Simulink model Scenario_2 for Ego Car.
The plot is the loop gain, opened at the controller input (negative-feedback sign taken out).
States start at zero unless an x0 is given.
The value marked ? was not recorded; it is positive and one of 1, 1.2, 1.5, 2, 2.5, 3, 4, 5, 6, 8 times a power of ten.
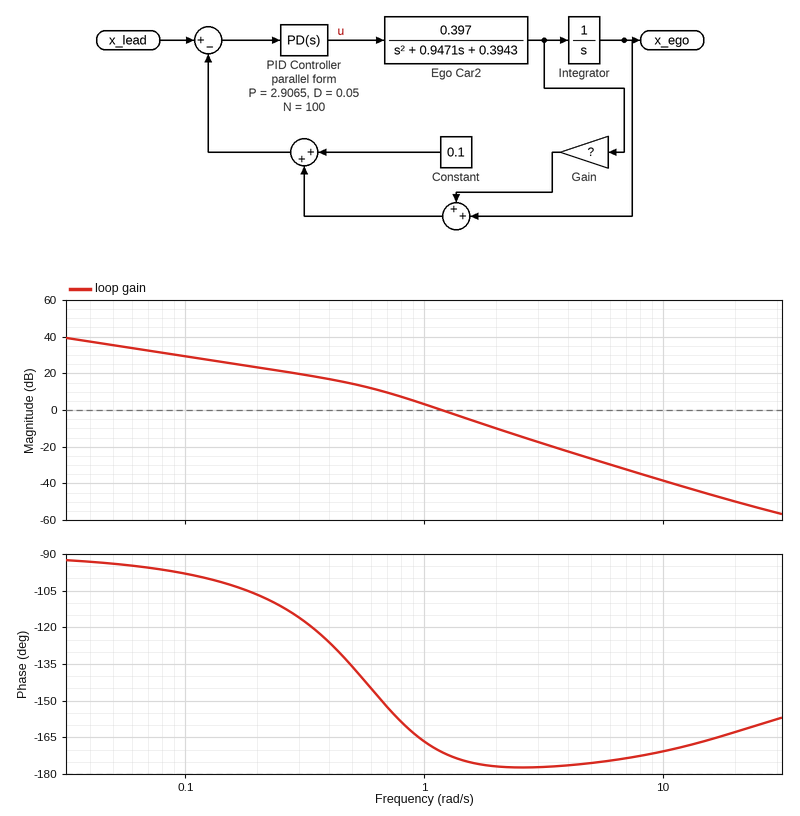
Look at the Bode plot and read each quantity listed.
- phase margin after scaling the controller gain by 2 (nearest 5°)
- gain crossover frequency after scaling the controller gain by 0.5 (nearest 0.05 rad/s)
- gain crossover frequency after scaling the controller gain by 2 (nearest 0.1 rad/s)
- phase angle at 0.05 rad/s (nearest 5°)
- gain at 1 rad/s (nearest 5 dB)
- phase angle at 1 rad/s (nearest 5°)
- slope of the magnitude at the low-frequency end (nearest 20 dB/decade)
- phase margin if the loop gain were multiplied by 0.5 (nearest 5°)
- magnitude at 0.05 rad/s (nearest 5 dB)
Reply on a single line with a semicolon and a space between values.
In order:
5°; 0.85 rad/s; 1.6 rad/s; -95°; 5 dB; -165°; -20 dB/decade; 20°; 35 dB
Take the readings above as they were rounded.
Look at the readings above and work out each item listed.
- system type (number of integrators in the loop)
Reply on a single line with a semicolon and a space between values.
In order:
1
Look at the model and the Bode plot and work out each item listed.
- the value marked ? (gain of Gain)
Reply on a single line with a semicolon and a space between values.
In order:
1
